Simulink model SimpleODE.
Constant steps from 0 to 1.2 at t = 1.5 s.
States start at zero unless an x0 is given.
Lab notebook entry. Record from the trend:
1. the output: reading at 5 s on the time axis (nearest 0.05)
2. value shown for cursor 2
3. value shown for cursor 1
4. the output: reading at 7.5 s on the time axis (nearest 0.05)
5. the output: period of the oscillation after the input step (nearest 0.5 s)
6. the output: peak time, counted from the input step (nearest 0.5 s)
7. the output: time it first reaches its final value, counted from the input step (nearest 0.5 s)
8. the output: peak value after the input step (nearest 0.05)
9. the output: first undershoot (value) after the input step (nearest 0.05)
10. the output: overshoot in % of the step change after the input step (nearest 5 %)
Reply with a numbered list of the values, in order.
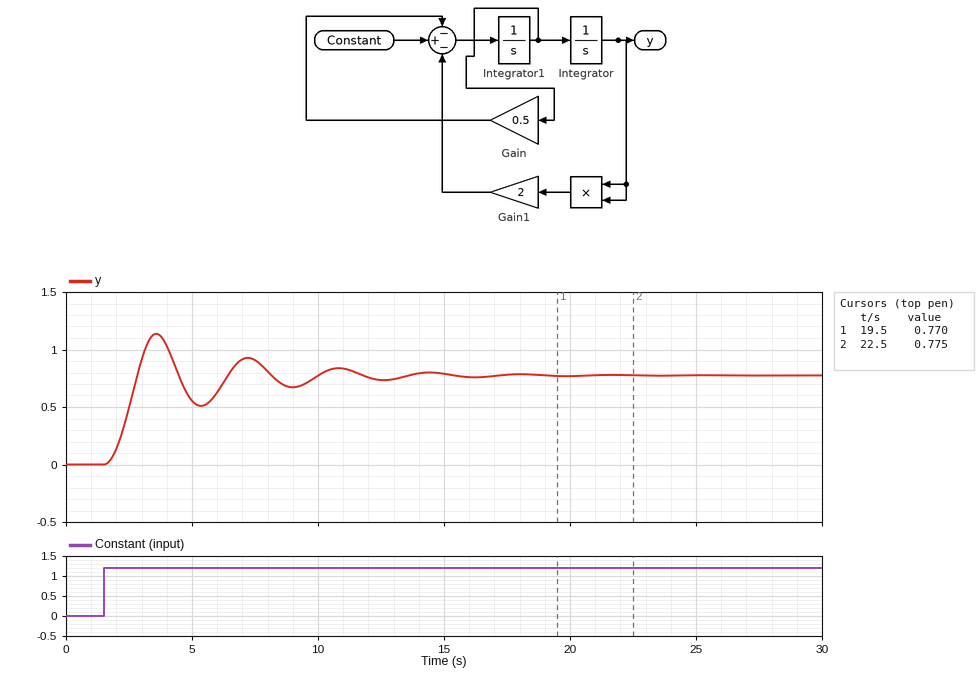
1. 0.55
2. 0.775
3. 0.770
4. 0.90
5. 3.5 s
6. 2.0 s
7. 1.5 s
8. 1.15
9. 0.50
10. 45 %
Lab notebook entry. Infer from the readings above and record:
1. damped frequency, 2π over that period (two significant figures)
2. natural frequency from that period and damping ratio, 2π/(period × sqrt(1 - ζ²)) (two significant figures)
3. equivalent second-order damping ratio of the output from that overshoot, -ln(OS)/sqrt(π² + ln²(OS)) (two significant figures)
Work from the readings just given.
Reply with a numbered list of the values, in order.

1. 1.8 rad/s
2. 1.9 rad/s
3. 0.25
